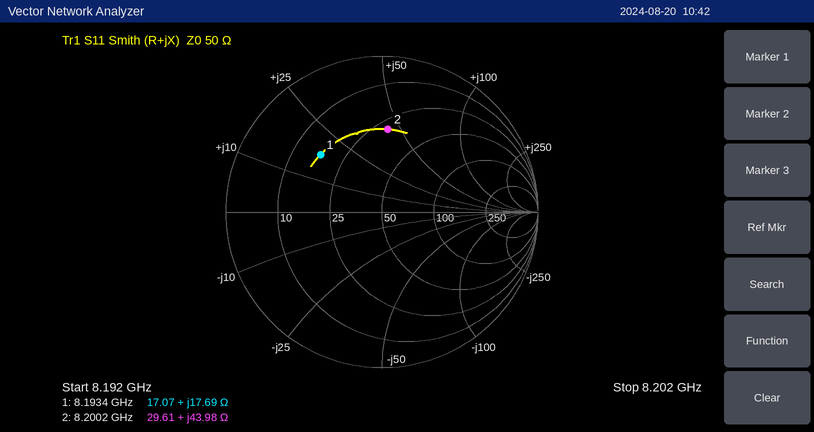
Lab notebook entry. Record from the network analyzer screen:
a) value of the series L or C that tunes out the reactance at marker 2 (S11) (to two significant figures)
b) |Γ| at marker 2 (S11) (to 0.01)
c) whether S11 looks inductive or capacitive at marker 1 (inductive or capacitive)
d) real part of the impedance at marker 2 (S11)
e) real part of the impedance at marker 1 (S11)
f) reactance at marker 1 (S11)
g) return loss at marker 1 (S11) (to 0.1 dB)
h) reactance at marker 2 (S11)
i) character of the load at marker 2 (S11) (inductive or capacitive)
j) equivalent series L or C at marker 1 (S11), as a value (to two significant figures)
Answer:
440 fF
0.53
inductive
29.61 Ω
17.07 Ω
+17.69 Ω
5.4 dB
+43.98 Ω
inductive
340 pH
